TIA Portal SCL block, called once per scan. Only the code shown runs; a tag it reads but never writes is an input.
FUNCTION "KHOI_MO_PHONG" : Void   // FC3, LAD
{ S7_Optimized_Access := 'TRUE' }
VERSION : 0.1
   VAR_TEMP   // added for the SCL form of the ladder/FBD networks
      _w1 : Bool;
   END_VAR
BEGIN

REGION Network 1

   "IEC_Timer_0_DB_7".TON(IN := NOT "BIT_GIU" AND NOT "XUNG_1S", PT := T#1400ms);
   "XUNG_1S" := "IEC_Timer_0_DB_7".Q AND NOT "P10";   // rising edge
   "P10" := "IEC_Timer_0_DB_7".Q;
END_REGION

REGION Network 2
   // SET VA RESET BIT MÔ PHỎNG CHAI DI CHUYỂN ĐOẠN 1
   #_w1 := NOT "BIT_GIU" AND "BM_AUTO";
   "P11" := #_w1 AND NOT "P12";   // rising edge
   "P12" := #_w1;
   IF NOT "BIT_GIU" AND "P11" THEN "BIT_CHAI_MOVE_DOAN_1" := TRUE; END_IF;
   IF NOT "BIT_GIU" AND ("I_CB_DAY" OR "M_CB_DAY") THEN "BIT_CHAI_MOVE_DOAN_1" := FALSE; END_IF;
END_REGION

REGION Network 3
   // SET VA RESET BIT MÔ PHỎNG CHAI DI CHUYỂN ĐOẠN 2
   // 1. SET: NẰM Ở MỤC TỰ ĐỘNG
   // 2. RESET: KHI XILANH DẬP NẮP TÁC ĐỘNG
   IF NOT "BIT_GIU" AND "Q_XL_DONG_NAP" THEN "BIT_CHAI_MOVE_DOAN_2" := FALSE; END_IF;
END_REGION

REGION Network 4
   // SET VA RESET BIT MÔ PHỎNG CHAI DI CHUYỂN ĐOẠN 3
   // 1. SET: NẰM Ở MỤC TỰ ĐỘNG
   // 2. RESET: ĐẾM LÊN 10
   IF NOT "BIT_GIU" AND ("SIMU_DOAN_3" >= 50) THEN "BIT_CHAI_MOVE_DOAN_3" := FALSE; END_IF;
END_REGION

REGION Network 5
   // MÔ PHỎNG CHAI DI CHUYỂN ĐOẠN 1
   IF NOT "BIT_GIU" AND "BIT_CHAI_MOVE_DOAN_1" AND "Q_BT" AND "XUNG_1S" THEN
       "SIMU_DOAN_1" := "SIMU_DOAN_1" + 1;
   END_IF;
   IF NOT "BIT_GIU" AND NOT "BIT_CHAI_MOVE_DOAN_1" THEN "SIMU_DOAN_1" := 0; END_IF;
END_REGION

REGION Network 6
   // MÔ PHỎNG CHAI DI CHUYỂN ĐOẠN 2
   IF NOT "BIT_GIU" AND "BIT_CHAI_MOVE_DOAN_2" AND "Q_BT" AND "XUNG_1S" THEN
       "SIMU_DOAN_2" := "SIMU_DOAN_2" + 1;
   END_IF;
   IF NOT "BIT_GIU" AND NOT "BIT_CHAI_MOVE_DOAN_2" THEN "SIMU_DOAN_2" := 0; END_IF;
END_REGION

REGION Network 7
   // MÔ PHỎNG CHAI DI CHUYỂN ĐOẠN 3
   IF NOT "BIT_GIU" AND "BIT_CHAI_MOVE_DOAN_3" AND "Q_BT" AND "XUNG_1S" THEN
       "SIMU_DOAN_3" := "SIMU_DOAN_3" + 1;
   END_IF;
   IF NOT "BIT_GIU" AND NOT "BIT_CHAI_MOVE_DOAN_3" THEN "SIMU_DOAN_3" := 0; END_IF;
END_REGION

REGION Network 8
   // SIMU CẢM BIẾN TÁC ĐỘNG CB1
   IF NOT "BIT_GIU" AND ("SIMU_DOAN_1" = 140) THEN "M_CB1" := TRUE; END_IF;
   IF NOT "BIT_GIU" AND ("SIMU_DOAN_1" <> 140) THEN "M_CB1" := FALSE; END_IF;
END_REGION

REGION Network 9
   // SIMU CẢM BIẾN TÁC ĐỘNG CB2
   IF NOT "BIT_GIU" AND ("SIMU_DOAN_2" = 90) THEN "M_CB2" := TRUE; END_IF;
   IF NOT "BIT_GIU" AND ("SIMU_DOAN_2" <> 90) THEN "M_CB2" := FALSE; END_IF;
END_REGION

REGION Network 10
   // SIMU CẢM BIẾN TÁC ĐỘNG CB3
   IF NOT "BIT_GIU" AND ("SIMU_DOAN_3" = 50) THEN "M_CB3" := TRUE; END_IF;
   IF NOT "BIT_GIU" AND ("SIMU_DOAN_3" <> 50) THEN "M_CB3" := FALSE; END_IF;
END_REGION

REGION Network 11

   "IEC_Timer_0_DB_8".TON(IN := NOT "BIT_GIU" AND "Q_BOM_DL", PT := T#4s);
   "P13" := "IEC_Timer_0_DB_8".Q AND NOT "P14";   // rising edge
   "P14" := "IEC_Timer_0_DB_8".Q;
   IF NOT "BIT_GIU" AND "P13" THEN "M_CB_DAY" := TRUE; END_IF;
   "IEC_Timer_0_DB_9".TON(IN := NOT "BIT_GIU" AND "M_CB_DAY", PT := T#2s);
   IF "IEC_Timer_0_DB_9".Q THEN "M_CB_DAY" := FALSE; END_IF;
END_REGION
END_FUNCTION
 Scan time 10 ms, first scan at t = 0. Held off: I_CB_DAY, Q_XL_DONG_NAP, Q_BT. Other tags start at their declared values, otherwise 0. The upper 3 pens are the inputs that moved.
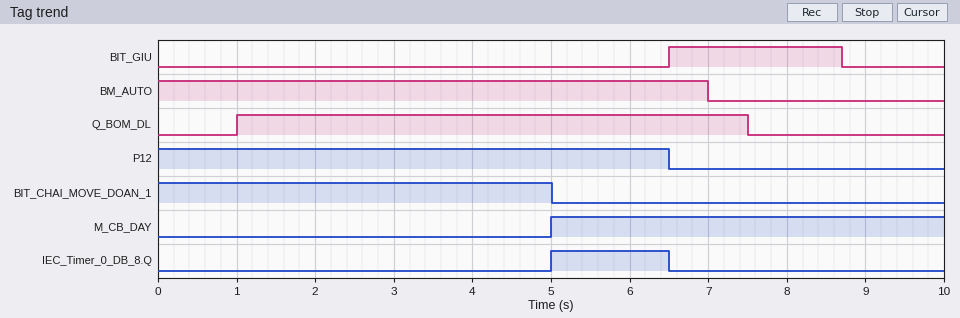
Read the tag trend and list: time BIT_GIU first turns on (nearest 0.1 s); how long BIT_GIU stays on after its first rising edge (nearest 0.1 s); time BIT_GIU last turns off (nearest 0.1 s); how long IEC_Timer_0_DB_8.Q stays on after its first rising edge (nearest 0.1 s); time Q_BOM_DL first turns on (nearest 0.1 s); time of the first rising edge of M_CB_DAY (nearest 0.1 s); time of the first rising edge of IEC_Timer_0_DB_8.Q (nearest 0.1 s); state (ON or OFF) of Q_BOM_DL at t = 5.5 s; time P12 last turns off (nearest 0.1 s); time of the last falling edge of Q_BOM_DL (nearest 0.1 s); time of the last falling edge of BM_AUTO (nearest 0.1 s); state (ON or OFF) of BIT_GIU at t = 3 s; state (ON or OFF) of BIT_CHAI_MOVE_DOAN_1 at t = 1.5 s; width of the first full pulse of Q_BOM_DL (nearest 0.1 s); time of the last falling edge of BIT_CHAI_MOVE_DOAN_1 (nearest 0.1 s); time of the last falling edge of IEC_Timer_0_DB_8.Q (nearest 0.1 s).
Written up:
6.5 s
2.2 s
8.7 s
1.5 s
1.0 s
5.0 s
5.0 s
ON
6.5 s
7.5 s
7.0 s
OFF
ON
6.5 s
5.0 s
6.5 s
